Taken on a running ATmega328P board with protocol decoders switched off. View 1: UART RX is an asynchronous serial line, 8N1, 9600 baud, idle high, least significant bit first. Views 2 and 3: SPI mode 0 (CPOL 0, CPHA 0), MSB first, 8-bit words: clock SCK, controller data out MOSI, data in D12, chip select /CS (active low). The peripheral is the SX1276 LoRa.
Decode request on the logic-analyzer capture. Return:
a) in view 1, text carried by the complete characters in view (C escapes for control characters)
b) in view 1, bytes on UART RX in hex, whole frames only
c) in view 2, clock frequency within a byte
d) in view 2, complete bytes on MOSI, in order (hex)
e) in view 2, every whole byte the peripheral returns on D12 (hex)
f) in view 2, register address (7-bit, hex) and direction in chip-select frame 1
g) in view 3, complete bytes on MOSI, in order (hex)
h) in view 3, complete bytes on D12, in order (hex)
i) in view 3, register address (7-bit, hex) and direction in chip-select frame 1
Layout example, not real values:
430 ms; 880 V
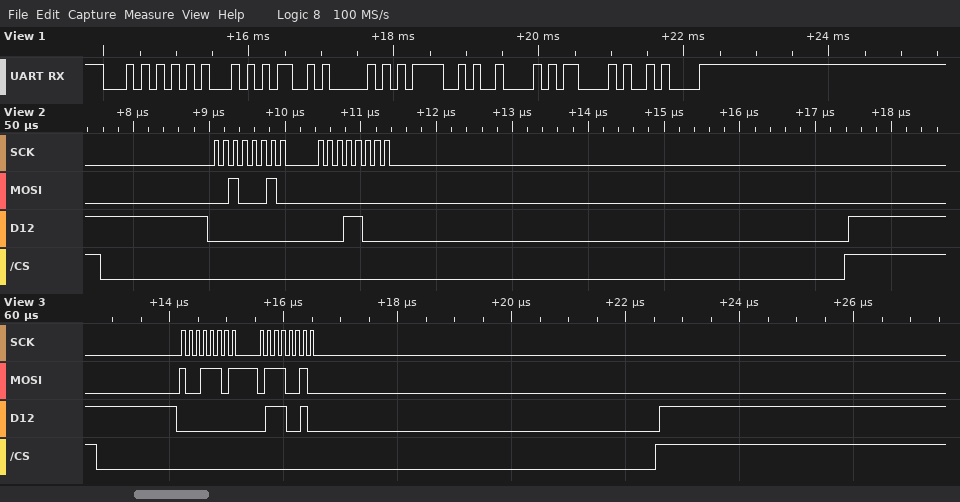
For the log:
"TEMPOBC\n"; 0x54 0x45 0x4D 0x50 0x4F 0x42 0x43 0x0A; 8 MHz; 22 00; 00 18; 0x22 read; 9D 72; 00 72; 0x1D write
